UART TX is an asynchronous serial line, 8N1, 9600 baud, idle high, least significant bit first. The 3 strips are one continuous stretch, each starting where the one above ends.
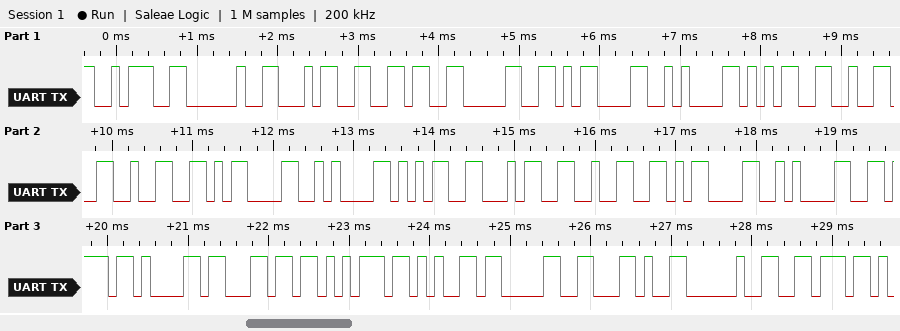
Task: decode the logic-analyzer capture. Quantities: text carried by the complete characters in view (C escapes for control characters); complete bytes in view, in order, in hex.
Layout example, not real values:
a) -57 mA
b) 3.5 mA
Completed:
a) ": 460\r\n522\r\n542\r\nvalue0, v"
b) 0x3A 0x20 0x34 0x36 0x30 0x0D 0x0A 0x35 0x32 0x32 0x0D 0x0A 0x35 0x34 0x32 0x0D 0x0A 0x76 0x61 0x6C 0x75 0x65 0x30 0x2C 0x20 0x76
